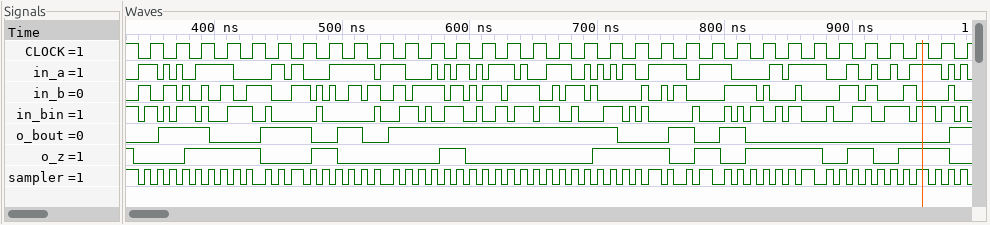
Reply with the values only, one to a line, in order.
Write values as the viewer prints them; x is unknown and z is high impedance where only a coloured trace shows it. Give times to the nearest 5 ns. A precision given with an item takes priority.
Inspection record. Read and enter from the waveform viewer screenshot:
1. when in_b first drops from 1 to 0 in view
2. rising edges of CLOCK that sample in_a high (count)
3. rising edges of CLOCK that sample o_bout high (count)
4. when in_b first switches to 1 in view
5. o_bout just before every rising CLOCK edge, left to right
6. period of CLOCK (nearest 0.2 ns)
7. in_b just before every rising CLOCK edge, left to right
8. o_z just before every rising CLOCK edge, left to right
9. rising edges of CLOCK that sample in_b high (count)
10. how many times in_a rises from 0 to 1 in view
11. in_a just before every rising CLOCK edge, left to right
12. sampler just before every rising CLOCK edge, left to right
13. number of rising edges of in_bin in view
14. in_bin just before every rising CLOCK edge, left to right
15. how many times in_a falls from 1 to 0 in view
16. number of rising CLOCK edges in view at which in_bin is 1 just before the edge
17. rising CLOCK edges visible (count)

350 ns
18
17
340 ns
0 1 1 0 0 1 1 0 1 0 1 1 1 1 1 1 1 1 1 0 0 1 0 1 0 0 0 0 0 0 0 0 1
20 ns
1 1 0 1 1 0 1 0 1 1 1 1 1 0 0 1 1 1 0 0 0 1 0 1 0 0 0 0 0 0 1 0 0
0 0 1 1 1 0 0 1 0 0 0 0 1 0 0 0 0 0 1 1 1 0 1 0 1 1 1 0 1 0 1 1 0
16
29
1 0 1 1 0 1 1 0 1 0 1 0 0 1 1 0 1 0 0 1 1 1 1 0 0 0 1 0 0 0 1 1 1
1 1 1 1 1 0 1 1 1 1 0 0 0 0 0 0 0 0 0 0 1 0 1 0 0 0 1 0 0 0 0 1 1
31
1 0 0 0 1 0 0 0 0 1 1 1 1 1 1 1 1 0 1 1 0 0 0 0 1 0 0 0 1 1 0 0 1
29
16
33
